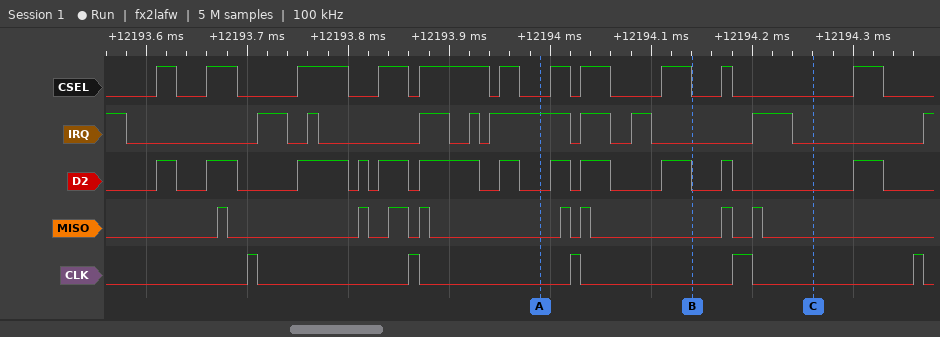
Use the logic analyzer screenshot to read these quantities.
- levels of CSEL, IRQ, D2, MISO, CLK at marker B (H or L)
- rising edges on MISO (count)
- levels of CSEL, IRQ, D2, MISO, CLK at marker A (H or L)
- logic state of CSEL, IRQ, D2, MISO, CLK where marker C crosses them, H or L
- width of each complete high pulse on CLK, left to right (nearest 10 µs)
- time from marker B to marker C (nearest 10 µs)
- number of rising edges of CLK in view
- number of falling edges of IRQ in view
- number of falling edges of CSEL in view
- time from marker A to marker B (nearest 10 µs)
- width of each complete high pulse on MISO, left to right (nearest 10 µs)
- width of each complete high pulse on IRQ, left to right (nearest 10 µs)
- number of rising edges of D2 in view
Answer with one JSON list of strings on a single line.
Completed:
["CSEL=L, IRQ=L, D2=L, MISO=L, CLK=L", "8", "CSEL=L, IRQ=H, D2=L, MISO=L, CLK=L", "CSEL=L, IRQ=L, D2=L, MISO=L, CLK=L", "10 µs, 10 µs, 10 µs, 20 µs, 10 µs", "120 µs", "5", "9", "11", "150 µs", "10 µs, 10 µs, 20 µs, 10 µs, 10 µs, 10 µs, 10 µs, 10 µs", "30 µs, 10 µs, 30 µs, 10 µs, 80 µs, 30 µs, 20 µs, 40 µs", "12"]
